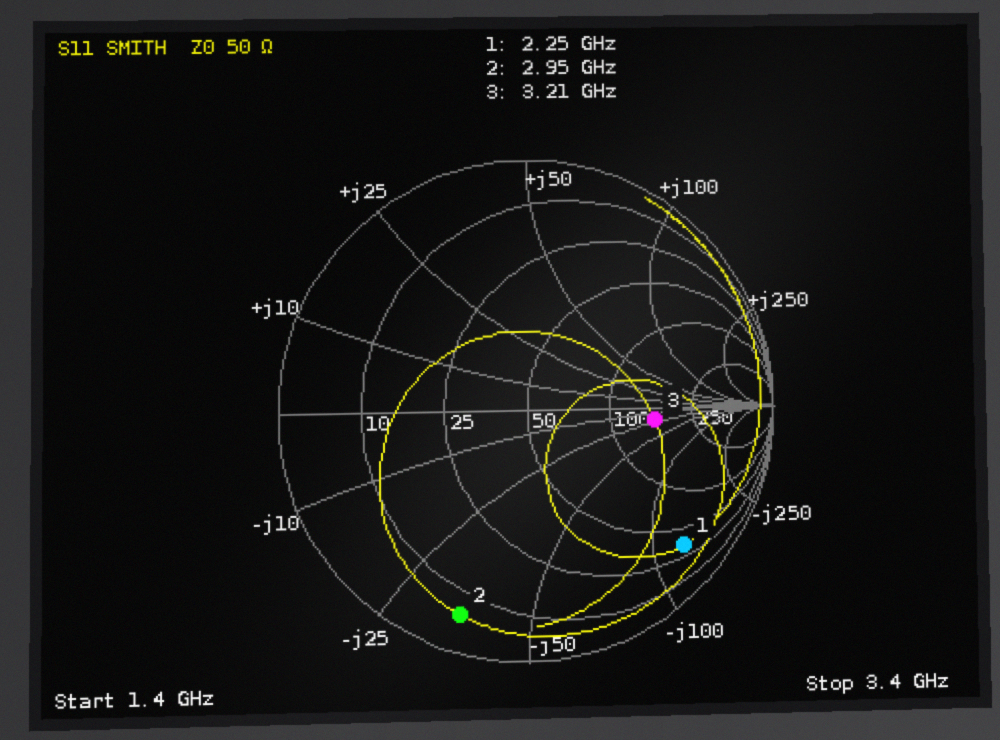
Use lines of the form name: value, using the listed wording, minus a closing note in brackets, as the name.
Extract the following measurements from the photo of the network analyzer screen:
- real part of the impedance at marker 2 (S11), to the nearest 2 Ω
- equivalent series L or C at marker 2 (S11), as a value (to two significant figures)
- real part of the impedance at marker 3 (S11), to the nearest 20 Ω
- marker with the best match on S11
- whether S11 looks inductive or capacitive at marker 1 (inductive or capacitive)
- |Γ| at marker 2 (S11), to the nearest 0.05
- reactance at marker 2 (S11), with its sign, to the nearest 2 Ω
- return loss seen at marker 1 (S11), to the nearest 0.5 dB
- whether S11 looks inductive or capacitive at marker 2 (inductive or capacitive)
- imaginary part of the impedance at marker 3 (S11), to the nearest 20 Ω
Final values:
real part of the impedance at marker 2 (S11), to the nearest 2 Ω: 6 Ω
equivalent series L or C at marker 2 (S11), as a value: 1.5 pF
real part of the impedance at marker 3 (S11), to the nearest 20 Ω: 160 Ω
marker with the best match on S11: marker 3
whether S11 looks inductive or capacitive at marker 1: capacitive
|Γ| at marker 2 (S11), to the nearest 0.05: 0.85
reactance at marker 2 (S11), with its sign, to the nearest 2 Ω: -36 Ω
return loss seen at marker 1 (S11), to the nearest 0.5 dB: 1.5 dB
whether S11 looks inductive or capacitive at marker 2: capacitive
imaginary part of the impedance at marker 3 (S11), to the nearest 20 Ω: -20 Ω
